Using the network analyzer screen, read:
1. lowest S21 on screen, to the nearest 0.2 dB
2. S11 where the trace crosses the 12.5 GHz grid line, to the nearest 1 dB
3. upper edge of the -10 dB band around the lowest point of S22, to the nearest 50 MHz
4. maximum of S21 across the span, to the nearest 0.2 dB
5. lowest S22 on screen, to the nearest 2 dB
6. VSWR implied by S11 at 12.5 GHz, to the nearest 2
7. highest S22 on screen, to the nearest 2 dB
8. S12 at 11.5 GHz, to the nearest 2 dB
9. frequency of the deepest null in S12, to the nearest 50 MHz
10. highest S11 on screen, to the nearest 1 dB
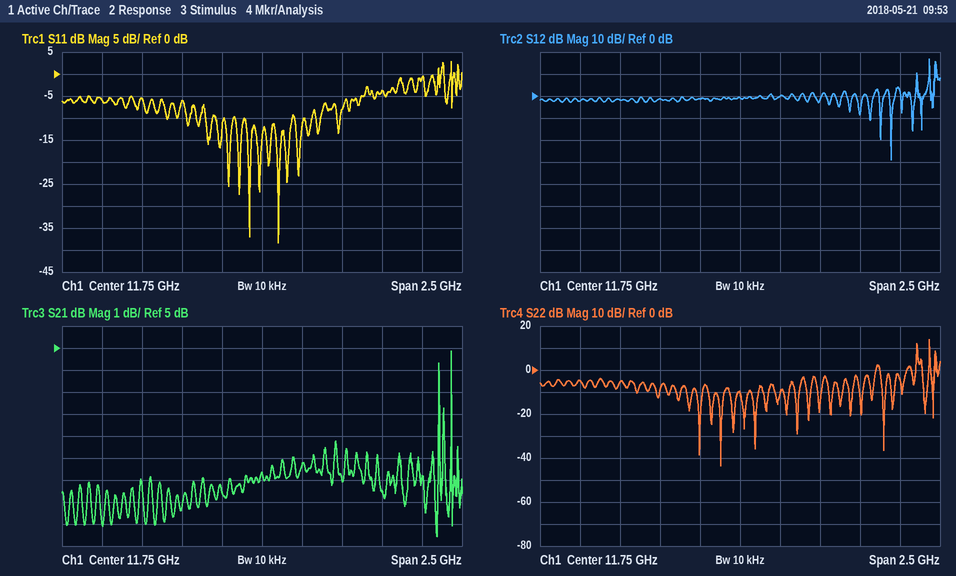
-3.6 dB
-4 dB
11.65 GHz
4.8 dB
-44 dB
4
14 dB
-2 dB
12.70 GHz
3 dB
